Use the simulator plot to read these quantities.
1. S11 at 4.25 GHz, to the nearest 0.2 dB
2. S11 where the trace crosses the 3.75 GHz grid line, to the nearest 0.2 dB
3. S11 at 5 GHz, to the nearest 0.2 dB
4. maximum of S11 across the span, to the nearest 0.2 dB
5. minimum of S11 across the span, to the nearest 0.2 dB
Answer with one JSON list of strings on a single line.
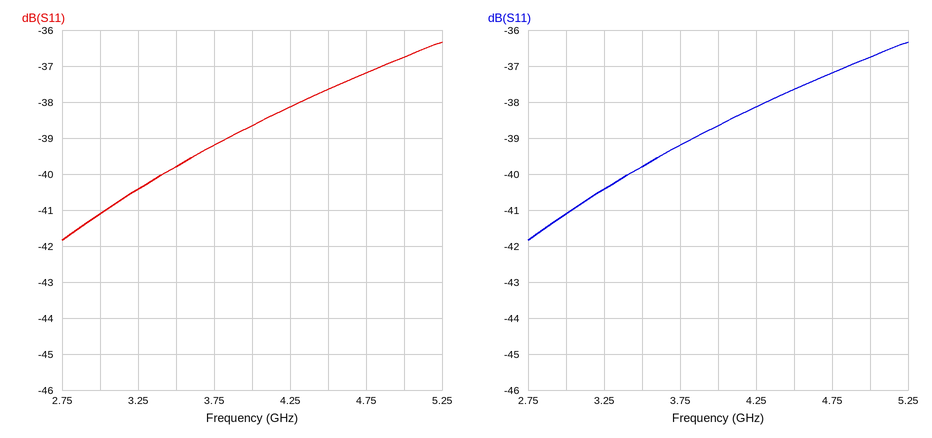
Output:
["-38.2 dB", "-39.2 dB", "-36.8 dB", "-36.4 dB", "-41.8 dB"]
